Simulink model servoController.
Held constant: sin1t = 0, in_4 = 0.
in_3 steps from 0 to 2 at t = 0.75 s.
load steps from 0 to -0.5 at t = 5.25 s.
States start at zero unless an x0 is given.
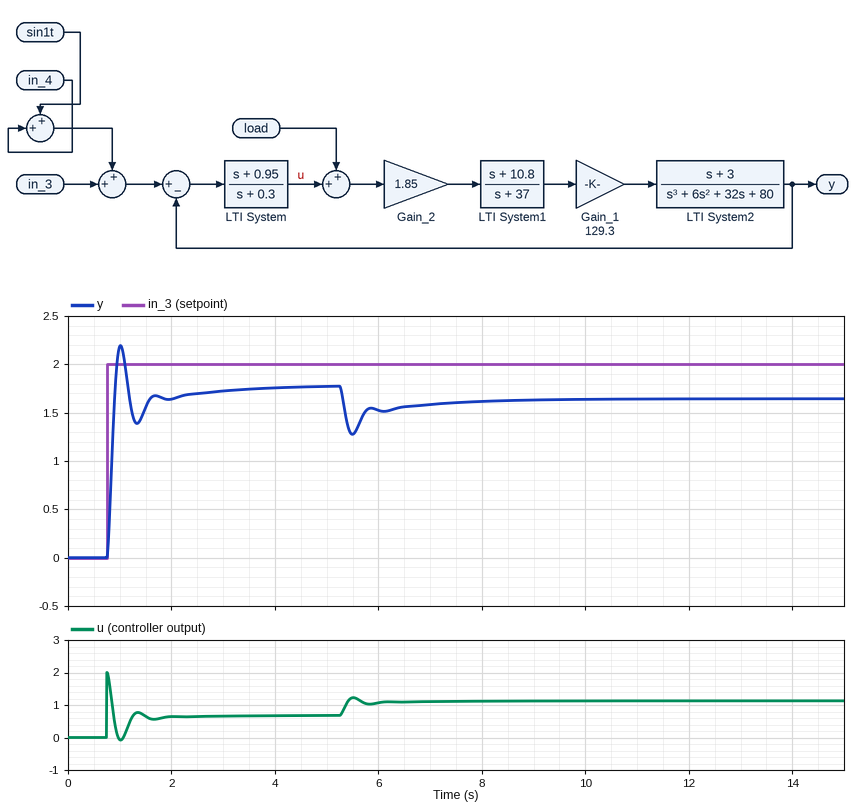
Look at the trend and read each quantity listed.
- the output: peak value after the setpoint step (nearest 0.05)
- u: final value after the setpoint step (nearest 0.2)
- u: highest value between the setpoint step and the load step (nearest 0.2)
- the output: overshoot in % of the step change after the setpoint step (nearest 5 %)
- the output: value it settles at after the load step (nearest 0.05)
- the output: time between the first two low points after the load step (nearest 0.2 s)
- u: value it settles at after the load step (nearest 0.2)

2.20
0.6
2.0
25 %
1.65
0.6 s
1.2
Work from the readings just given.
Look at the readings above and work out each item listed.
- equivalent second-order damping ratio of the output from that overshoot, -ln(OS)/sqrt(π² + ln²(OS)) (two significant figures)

0.40
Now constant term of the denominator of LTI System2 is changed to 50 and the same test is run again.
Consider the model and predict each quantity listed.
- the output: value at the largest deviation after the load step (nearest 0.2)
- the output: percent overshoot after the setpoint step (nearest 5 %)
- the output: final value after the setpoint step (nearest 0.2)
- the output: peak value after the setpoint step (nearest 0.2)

1.4
20 %
1.8
2.2
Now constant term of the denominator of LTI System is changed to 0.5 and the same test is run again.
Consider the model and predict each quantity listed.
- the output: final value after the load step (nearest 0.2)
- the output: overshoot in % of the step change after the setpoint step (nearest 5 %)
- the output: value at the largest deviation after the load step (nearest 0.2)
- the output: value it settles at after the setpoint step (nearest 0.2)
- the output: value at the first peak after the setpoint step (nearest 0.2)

1.4
30 %
1.2
1.6
2.2
